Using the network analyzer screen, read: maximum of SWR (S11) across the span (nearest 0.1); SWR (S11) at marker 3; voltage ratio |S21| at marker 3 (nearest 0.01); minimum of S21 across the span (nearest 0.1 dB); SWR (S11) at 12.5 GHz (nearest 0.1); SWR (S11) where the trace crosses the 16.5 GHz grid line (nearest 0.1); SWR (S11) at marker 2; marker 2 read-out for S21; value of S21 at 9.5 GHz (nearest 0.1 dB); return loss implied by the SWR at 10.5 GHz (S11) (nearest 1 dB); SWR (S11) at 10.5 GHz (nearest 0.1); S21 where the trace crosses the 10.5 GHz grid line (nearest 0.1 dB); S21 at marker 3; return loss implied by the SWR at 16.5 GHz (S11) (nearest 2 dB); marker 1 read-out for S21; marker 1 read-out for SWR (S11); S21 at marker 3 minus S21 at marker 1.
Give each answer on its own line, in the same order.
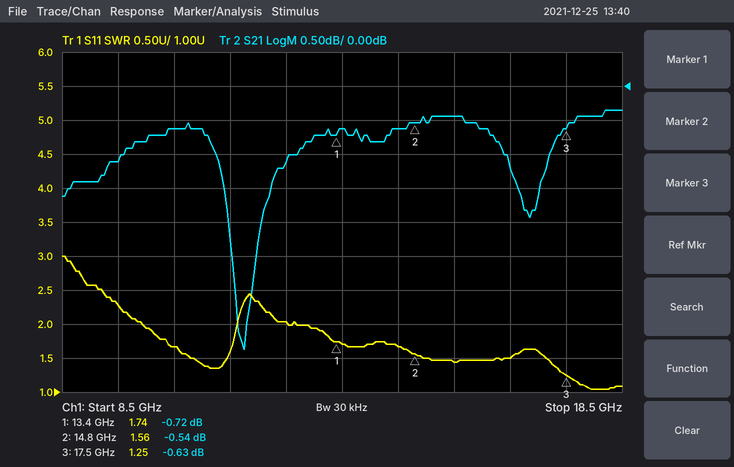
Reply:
3.0
1.25
0.93
-3.9 dB
2.0
1.5
1.56
-0.54 dB
-1.1 dB
12 dB
1.7
-0.6 dB
-0.63 dB
14 dB
-0.72 dB
1.74
0.09 dB
